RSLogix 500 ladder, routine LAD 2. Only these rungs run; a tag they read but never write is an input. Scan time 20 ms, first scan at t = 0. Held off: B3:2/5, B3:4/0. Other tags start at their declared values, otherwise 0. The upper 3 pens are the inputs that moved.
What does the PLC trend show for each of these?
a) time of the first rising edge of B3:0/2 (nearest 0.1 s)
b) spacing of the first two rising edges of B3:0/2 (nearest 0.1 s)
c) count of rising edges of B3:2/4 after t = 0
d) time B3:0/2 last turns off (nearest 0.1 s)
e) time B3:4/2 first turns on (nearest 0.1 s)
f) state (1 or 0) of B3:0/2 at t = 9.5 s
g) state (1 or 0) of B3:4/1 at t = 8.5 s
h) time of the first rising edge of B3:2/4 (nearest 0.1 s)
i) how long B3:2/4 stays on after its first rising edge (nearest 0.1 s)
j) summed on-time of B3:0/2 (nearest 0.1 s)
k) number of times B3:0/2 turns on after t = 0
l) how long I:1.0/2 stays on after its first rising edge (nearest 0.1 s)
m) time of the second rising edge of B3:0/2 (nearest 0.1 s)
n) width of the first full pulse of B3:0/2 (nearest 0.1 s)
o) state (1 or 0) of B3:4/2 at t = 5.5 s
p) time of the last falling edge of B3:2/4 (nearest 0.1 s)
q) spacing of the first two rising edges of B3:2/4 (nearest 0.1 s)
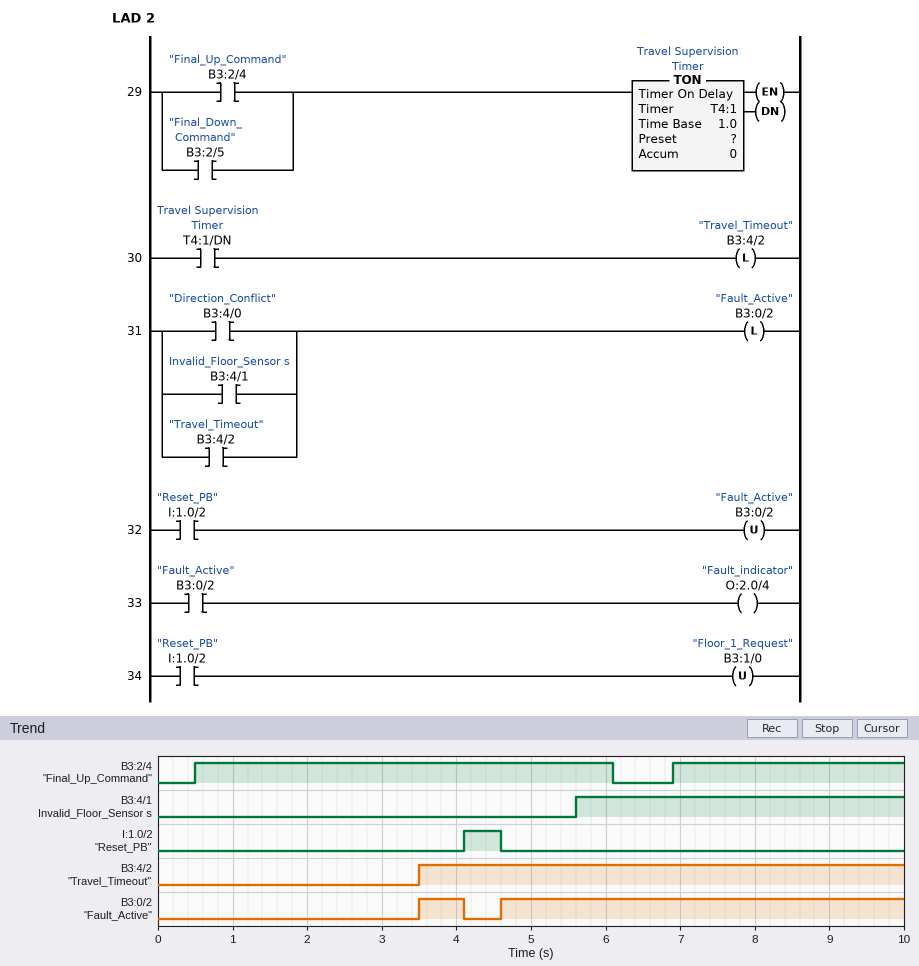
3.5 s
1.1 s
2
4.1 s
3.5 s
1
1
0.5 s
5.6 s
6.0 s
2
0.5 s
4.6 s
0.6 s
1
6.1 s
6.4 s
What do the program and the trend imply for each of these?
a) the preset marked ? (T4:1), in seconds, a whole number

3 s
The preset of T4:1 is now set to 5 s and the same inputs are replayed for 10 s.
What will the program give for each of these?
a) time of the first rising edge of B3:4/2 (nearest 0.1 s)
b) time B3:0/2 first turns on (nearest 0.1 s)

5.5 s
5.5 s
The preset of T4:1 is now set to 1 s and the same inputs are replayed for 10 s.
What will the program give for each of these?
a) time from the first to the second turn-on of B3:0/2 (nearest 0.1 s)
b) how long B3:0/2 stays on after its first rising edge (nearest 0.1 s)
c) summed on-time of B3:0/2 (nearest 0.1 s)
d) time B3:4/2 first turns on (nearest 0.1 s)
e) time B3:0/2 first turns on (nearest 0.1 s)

3.1 s
2.6 s
8.0 s
1.5 s
1.5 s
